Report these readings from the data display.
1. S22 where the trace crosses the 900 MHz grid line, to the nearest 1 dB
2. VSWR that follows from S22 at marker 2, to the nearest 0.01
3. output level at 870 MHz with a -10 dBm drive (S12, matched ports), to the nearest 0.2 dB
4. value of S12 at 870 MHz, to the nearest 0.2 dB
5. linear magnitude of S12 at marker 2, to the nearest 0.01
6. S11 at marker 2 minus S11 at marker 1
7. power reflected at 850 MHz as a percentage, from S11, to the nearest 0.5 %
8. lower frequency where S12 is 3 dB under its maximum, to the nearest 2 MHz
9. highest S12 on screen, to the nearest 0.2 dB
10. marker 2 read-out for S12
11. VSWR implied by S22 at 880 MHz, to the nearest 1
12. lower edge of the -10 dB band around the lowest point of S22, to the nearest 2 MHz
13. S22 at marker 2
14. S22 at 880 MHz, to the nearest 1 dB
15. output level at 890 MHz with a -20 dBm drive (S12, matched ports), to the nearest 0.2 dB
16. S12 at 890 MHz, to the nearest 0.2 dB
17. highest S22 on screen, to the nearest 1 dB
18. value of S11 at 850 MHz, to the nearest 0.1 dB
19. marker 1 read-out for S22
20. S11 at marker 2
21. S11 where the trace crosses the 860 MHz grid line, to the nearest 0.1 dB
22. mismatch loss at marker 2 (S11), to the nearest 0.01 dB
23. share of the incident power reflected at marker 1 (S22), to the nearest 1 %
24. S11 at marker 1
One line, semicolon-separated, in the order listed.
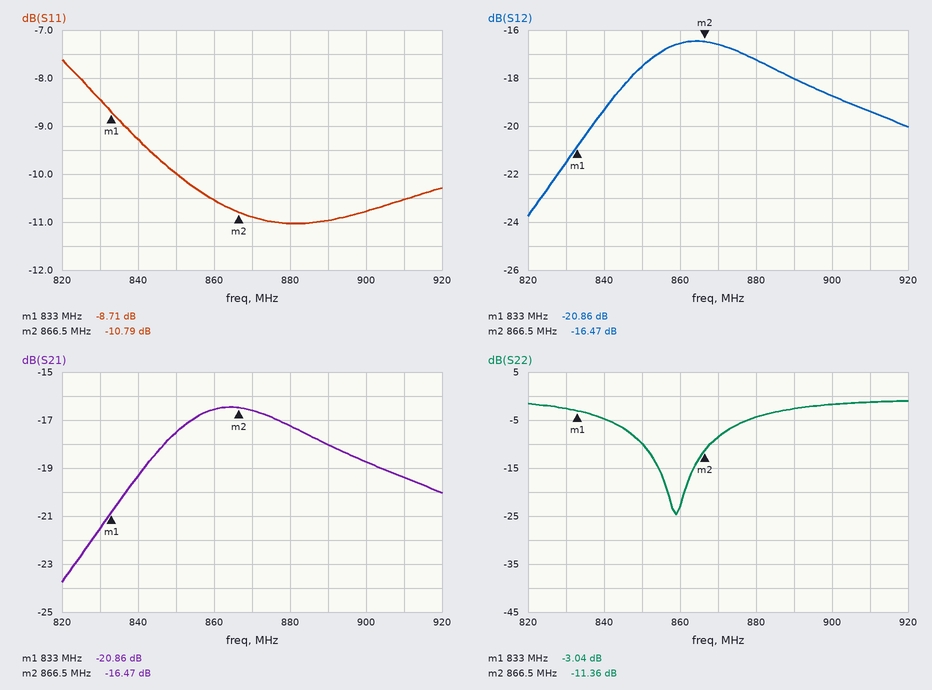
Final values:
-2 dB; 1.74; -26.6 dBm; -16.6 dB; 0.15; -2.08 dB; 10.0 %; 840 MHz; -16.4 dB; -16.47 dB; 4; 850 MHz; -11.36 dB; -4 dB; -38.0 dBm; -18.0 dB; -1 dB; -10.0 dB; -3.04 dB; -10.79 dB; -10.5 dB; 0.38 dB; 50 %; -8.71 dB
